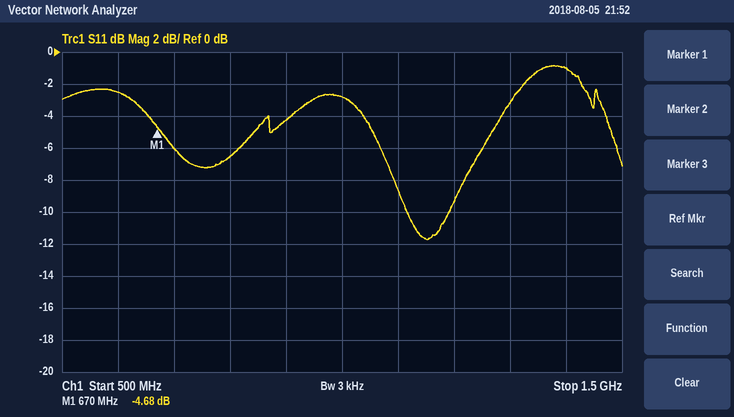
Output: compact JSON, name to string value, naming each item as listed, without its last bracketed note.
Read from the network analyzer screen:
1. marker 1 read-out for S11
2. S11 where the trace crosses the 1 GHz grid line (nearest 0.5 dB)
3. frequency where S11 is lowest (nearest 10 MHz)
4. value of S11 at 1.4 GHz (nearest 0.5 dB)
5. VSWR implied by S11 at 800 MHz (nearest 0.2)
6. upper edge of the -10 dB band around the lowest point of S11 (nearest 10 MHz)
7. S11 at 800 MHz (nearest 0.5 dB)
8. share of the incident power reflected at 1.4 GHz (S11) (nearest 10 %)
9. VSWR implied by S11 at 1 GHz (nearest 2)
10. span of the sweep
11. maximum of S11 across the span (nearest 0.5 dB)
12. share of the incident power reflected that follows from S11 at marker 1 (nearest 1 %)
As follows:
{"marker 1 read-out for S11": "-4.68 dB", "S11 where the trace crosses the 1 GHz grid line": "-3.0 dB", "frequency where S11 is lowest": "1.15 GHz", "value of S11 at 1.4 GHz": "-1.0 dB", "VSWR implied by S11 at 800 MHz": "2.8", "upper edge of the -10 dB band around the lowest point of S11": "1.19 GHz", "S11 at 800 MHz": "-6.5 dB", "share of the incident power reflected at 1.4 GHz (S11)": "80 %", "VSWR implied by S11 at 1 GHz": "6", "span of the sweep": "1 GHz", "maximum of S11 across the span": "-1.0 dB", "share of the incident power reflected that follows from S11 at marker 1": "34 %"}
